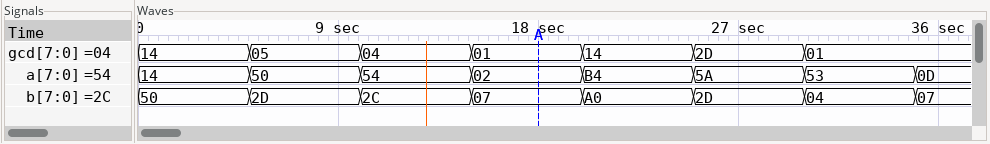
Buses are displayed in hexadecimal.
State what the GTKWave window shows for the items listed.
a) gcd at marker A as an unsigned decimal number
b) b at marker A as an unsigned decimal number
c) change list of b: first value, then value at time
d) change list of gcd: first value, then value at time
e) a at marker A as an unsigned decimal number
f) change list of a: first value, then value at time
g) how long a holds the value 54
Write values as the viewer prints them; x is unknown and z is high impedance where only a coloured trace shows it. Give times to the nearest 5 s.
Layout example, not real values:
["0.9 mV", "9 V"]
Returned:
["1", "7", "50, 2D at 5 s, 2C at 10 s, 07 at 15 s, A0 at 20 s, 2D at 25 s, 04 at 30 s, 07 at 35 s", "14, 05 at 5 s, 04 at 10 s, 01 at 15 s, 14 at 20 s, 2D at 25 s, 01 at 30 s", "2", "14, 50 at 5 s, 54 at 10 s, 02 at 15 s, B4 at 20 s, 5A at 25 s, 53 at 30 s, 0D at 35 s", "5 s"]
